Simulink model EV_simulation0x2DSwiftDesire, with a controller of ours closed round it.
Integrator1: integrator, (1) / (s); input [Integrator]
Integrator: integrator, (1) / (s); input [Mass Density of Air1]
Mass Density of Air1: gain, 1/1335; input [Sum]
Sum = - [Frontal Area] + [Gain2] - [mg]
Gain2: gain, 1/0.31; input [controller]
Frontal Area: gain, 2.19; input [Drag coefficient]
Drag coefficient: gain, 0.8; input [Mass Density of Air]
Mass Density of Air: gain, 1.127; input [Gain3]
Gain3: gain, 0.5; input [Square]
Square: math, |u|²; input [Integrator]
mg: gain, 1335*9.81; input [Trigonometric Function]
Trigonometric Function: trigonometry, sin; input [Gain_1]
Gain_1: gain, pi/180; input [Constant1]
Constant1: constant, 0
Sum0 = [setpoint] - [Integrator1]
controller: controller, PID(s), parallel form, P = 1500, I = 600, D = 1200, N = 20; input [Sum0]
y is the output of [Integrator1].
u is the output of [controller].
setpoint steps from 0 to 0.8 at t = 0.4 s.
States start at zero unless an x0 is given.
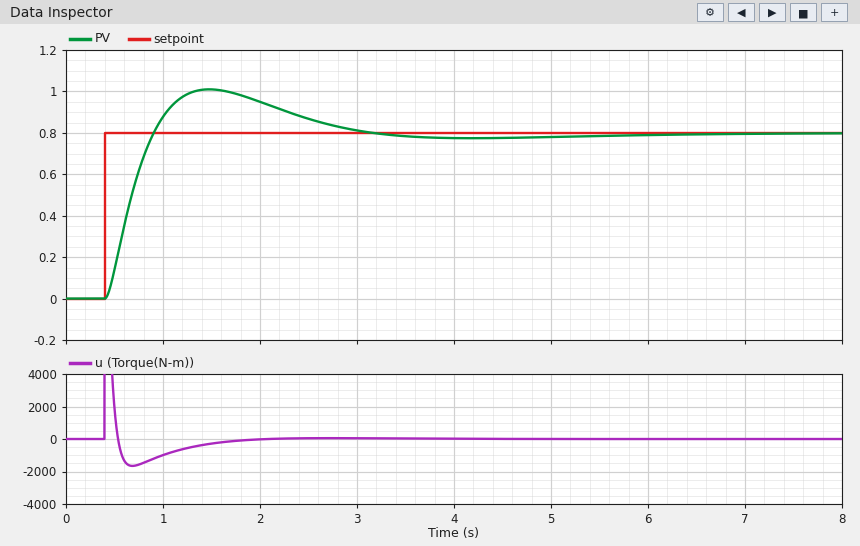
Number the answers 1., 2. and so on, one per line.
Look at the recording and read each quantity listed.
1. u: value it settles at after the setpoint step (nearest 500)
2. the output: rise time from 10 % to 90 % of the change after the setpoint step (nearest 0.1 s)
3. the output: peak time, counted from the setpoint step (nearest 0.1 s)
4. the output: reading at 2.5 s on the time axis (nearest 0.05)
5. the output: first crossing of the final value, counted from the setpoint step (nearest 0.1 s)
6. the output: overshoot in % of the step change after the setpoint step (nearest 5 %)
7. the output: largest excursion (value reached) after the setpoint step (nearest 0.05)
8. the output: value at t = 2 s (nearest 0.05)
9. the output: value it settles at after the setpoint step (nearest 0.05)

1. 0
2. 0.4 s
3. 1.1 s
4. 0.85
5. 0.5 s
6. 25 %
7. 1.00
8. 0.95
9. 0.80
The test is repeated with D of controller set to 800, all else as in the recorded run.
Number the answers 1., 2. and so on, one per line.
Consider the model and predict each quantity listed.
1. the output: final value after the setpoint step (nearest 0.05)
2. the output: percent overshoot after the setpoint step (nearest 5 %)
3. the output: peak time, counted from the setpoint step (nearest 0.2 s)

1. 0.80
2. 40 %
3. 1.2 s
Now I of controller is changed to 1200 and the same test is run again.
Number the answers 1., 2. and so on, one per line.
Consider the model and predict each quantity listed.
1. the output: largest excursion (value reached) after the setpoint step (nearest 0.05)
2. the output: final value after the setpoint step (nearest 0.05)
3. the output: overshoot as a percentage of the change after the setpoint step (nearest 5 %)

1. 1.05
2. 0.80
3. 30 %
